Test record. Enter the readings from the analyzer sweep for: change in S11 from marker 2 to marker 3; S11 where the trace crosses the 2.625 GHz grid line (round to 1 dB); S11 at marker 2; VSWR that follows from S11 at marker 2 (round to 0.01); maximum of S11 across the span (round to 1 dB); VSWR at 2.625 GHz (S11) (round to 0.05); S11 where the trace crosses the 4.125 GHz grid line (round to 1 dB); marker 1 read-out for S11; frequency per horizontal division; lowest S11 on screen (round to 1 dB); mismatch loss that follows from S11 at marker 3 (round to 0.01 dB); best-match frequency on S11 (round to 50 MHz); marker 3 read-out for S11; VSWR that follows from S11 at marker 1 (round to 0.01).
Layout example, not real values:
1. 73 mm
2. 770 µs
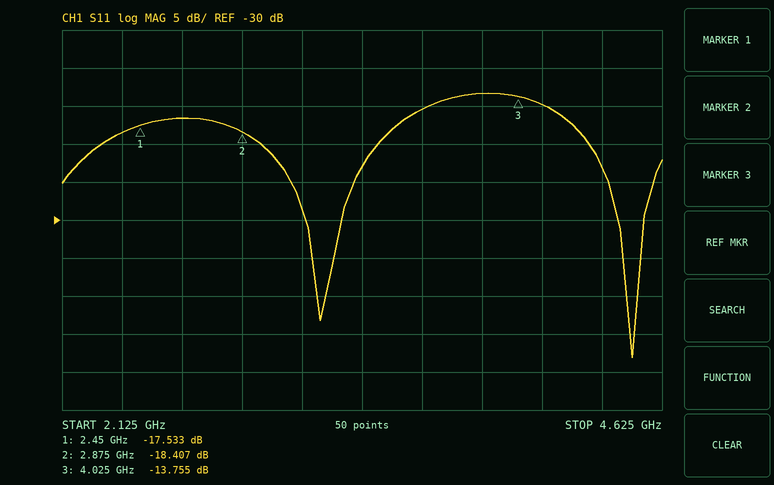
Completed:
1. 4.652 dB
2. -17 dB
3. -18.407 dB
4. 1.27
5. -13 dB
6. 1.35
7. -15 dB
8. -17.533 dB
9. 250 MHz
10. -48 dB
11. 0.19 dB
12. 4.50 GHz
13. -13.755 dB
14. 1.31
